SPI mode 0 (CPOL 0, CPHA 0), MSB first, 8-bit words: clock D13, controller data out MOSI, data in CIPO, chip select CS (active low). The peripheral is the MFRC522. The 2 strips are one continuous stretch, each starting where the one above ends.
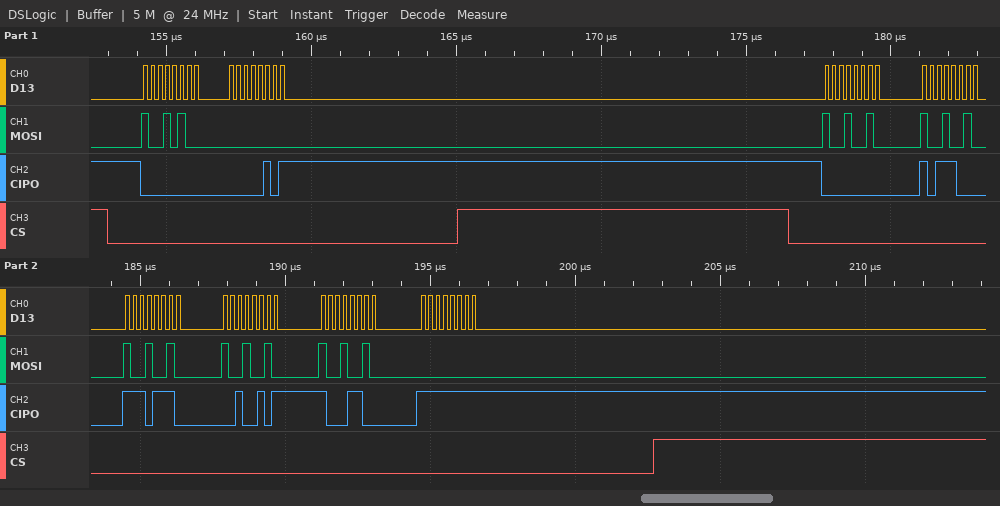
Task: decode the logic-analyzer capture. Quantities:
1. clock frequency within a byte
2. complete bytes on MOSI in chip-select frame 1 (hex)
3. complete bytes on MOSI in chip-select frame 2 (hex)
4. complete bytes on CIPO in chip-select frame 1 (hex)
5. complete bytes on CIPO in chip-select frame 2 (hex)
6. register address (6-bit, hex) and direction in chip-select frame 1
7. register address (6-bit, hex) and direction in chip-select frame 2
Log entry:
4 MHz
94 00
92 92 92 92 92 00
00 05
00 B8 EE 25 8C FF
0x0A read
0x09 read
